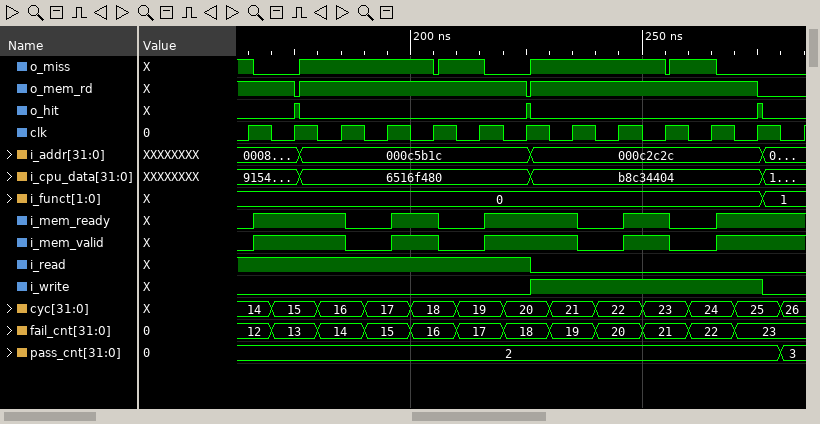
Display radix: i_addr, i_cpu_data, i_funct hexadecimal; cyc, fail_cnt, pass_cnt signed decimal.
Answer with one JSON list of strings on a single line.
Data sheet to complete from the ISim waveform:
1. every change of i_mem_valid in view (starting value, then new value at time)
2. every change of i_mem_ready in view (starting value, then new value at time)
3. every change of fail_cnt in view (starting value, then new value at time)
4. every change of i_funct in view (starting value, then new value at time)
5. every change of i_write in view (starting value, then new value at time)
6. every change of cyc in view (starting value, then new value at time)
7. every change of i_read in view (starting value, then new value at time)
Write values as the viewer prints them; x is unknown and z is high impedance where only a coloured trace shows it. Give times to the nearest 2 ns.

["0, 1 at 166 ns, 0 at 186 ns, 1 at 196 ns, 0 at 206 ns, 1 at 216 ns, 0 at 236 ns, 1 at 246 ns, 0 at 256 ns, 1 at 266 ns", "0, 1 at 166 ns, 0 at 186 ns, 1 at 196 ns, 0 at 206 ns, 1 at 216 ns, 0 at 236 ns, 1 at 246 ns, 0 at 256 ns, 1 at 266 ns", "12, 13 at 170 ns, 14 at 180 ns, 15 at 190 ns, 16 at 200 ns, 17 at 210 ns, 18 at 220 ns, 19 at 230 ns, 20 at 240 ns, 21 at 250 ns, 22 at 260 ns, 23 at 270 ns", "0, 1 at 276 ns", "0, 1 at 226 ns, 0 at 276 ns", "14, 15 at 170 ns, 16 at 180 ns, 17 at 190 ns, 18 at 200 ns, 19 at 210 ns, 20 at 220 ns, 21 at 230 ns, 22 at 240 ns, 23 at 250 ns, 24 at 260 ns, 25 at 270 ns, 26 at 280 ns", "1, 0 at 226 ns"]
